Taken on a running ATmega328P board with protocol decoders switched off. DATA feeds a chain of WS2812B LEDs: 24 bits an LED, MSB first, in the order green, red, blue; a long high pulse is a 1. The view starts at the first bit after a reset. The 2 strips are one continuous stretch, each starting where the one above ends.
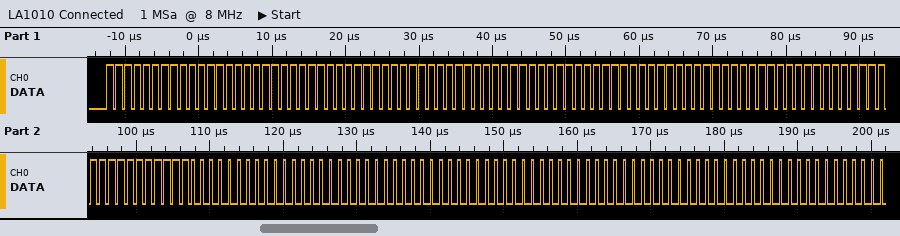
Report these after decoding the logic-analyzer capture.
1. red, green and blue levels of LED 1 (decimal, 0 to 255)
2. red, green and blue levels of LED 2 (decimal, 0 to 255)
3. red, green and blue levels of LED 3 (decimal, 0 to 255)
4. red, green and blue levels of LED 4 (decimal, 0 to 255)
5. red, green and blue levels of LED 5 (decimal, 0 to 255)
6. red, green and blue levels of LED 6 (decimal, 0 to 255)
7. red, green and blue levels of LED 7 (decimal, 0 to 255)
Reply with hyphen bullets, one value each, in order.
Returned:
- 255, 255, 255
- 255, 255, 255
- 255, 255, 255
- 255, 255, 255
- 0, 0, 0
- 0, 0, 0
- 0, 0, 0
